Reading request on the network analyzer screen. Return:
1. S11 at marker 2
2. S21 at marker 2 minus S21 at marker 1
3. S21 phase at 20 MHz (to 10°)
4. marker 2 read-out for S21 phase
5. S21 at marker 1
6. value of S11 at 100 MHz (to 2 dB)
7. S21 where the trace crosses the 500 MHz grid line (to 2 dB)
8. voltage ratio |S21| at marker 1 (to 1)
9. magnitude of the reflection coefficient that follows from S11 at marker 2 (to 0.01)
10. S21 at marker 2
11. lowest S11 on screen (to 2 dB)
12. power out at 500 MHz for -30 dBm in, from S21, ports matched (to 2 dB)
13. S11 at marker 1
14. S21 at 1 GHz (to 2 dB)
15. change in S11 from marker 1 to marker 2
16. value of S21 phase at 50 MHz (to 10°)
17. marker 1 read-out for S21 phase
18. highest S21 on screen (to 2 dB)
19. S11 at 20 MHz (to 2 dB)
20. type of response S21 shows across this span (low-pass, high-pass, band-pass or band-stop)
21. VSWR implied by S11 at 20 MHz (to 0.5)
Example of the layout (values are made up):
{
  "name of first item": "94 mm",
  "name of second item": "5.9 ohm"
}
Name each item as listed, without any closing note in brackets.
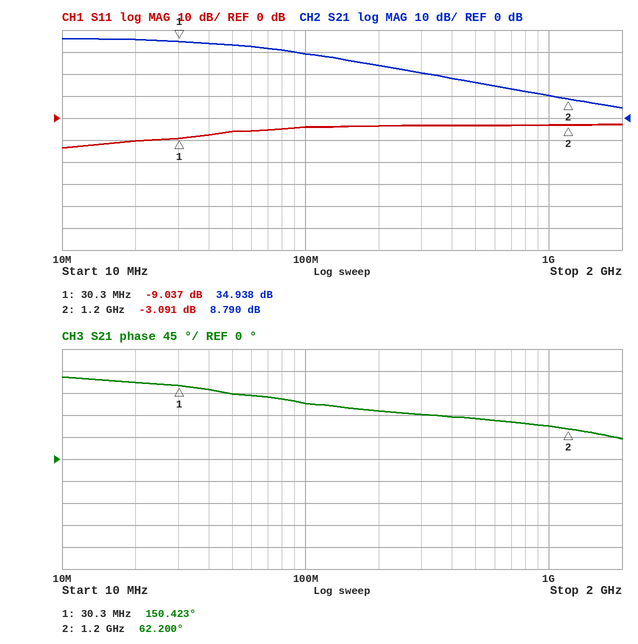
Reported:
{
  "S11 at marker 2": "-3.091 dB",
  "S21 at marker 2 minus S21 at marker 1": "-26.148 dB",
  "S21 phase at 20 MHz": "160°",
  "marker 2 read-out for S21 phase": "62.200°",
  "S21 at marker 1": "34.938 dB",
  "value of S11 at 100 MHz": "-4 dB",
  "S21 where the trace crosses the 500 MHz grid line": "16 dB",
  "voltage ratio |S21| at marker 1": "56",
  "magnitude of the reflection coefficient that follows from S11 at marker 2": "0.70",
  "S21 at marker 2": "8.790 dB",
  "lowest S11 on screen": "-14 dB",
  "power out at 500 MHz for -30 dBm in, from S21, ports matched": "-14 dBm",
  "S11 at marker 1": "-9.037 dB",
  "S21 at 1 GHz": "10 dB",
  "change in S11 from marker 1 to marker 2": "5.946 dB",
  "value of S21 phase at 50 MHz": "130°",
  "marker 1 read-out for S21 phase": "150.423°",
  "highest S21 on screen": "36 dB",
  "S11 at 20 MHz": "-10 dB",
  "type of response S21 shows across this span": "low-pass",
  "VSWR implied by S11 at 20 MHz": "2.0"
}
